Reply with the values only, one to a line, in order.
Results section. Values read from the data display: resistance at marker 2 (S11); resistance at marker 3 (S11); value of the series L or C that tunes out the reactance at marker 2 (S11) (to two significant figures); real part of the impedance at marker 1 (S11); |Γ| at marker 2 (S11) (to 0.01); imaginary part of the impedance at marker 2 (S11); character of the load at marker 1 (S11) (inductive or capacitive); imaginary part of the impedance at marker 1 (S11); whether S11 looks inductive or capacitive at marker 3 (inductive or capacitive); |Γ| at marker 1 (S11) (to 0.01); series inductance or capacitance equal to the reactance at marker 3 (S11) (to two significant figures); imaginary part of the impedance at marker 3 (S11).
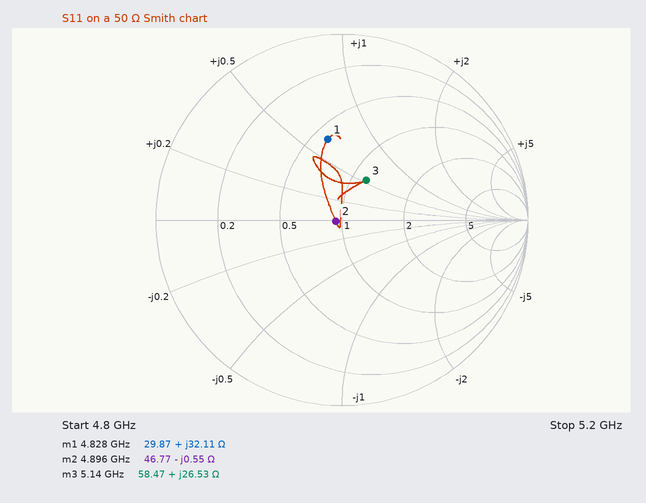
46.77 Ω
58.47 Ω
18 pH
29.87 Ω
0.03
-0.55 Ω
inductive
+32.11 Ω
inductive
0.44
820 pH
+26.53 Ω
